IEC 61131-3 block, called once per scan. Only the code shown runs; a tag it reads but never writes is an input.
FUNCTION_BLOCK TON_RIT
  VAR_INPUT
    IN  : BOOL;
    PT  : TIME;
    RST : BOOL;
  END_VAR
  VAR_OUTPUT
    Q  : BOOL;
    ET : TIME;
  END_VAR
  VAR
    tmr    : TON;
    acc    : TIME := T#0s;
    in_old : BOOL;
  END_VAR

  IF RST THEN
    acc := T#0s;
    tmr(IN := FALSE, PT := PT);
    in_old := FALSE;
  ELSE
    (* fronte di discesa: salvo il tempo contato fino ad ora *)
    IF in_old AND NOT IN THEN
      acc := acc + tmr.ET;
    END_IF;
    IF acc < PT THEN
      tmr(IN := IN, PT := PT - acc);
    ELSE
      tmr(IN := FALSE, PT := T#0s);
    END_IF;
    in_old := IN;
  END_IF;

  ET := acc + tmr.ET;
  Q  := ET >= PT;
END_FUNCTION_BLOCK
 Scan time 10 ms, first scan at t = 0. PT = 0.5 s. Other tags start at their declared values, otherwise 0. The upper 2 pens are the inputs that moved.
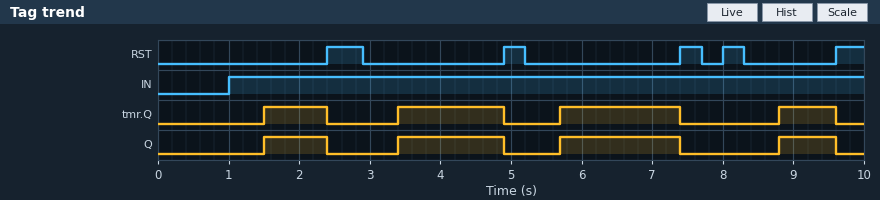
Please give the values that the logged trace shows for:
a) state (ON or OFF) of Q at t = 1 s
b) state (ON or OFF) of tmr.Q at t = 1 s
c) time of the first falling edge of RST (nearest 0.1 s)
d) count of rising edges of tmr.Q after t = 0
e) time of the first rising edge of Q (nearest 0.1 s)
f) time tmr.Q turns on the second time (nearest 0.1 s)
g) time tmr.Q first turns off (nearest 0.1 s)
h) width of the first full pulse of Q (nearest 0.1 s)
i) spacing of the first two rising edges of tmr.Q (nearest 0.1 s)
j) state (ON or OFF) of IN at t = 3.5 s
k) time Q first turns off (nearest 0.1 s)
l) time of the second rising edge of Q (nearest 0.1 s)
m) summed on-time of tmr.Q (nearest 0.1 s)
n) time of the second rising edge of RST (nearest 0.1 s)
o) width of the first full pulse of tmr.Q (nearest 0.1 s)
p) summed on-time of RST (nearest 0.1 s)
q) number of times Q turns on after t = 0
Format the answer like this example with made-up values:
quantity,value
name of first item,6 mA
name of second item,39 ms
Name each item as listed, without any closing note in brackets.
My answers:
quantity,value
state (ON or OFF) of Q at t = 1 s,OFF
state (ON or OFF) of tmr.Q at t = 1 s,OFF
time of the first falling edge of RST,2.9 s
count of rising edges of tmr.Q after t = 0,4
time of the first rising edge of Q,1.5 s
time tmr.Q turns on the second time,3.4 s
time tmr.Q first turns off,2.4 s
width of the first full pulse of Q,0.9 s
spacing of the first two rising edges of tmr.Q,1.9 s
state (ON or OFF) of IN at t = 3.5 s,ON
time Q first turns off,2.4 s
time of the second rising edge of Q,3.4 s
summed on-time of tmr.Q,4.9 s
time of the second rising edge of RST,4.9 s
width of the first full pulse of tmr.Q,0.9 s
summed on-time of RST,1.8 s
number of times Q turns on after t = 0,4
